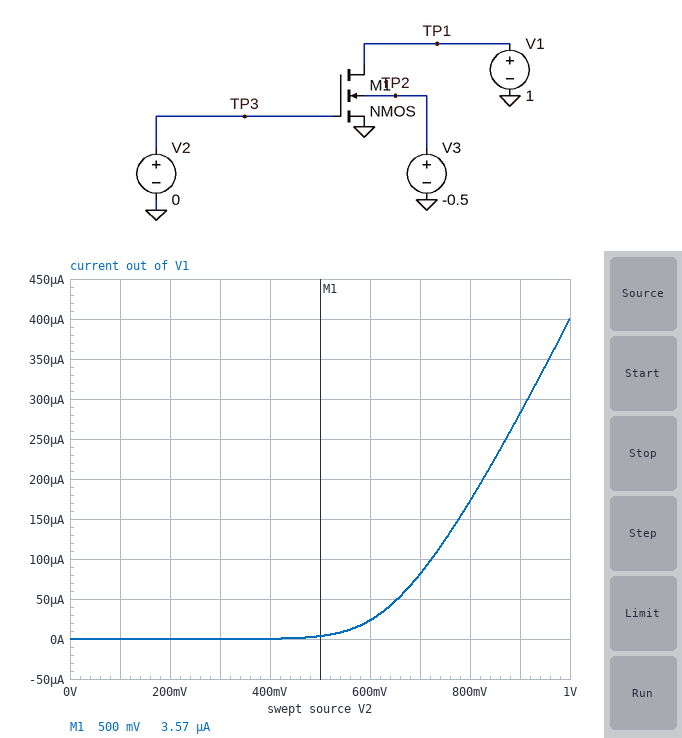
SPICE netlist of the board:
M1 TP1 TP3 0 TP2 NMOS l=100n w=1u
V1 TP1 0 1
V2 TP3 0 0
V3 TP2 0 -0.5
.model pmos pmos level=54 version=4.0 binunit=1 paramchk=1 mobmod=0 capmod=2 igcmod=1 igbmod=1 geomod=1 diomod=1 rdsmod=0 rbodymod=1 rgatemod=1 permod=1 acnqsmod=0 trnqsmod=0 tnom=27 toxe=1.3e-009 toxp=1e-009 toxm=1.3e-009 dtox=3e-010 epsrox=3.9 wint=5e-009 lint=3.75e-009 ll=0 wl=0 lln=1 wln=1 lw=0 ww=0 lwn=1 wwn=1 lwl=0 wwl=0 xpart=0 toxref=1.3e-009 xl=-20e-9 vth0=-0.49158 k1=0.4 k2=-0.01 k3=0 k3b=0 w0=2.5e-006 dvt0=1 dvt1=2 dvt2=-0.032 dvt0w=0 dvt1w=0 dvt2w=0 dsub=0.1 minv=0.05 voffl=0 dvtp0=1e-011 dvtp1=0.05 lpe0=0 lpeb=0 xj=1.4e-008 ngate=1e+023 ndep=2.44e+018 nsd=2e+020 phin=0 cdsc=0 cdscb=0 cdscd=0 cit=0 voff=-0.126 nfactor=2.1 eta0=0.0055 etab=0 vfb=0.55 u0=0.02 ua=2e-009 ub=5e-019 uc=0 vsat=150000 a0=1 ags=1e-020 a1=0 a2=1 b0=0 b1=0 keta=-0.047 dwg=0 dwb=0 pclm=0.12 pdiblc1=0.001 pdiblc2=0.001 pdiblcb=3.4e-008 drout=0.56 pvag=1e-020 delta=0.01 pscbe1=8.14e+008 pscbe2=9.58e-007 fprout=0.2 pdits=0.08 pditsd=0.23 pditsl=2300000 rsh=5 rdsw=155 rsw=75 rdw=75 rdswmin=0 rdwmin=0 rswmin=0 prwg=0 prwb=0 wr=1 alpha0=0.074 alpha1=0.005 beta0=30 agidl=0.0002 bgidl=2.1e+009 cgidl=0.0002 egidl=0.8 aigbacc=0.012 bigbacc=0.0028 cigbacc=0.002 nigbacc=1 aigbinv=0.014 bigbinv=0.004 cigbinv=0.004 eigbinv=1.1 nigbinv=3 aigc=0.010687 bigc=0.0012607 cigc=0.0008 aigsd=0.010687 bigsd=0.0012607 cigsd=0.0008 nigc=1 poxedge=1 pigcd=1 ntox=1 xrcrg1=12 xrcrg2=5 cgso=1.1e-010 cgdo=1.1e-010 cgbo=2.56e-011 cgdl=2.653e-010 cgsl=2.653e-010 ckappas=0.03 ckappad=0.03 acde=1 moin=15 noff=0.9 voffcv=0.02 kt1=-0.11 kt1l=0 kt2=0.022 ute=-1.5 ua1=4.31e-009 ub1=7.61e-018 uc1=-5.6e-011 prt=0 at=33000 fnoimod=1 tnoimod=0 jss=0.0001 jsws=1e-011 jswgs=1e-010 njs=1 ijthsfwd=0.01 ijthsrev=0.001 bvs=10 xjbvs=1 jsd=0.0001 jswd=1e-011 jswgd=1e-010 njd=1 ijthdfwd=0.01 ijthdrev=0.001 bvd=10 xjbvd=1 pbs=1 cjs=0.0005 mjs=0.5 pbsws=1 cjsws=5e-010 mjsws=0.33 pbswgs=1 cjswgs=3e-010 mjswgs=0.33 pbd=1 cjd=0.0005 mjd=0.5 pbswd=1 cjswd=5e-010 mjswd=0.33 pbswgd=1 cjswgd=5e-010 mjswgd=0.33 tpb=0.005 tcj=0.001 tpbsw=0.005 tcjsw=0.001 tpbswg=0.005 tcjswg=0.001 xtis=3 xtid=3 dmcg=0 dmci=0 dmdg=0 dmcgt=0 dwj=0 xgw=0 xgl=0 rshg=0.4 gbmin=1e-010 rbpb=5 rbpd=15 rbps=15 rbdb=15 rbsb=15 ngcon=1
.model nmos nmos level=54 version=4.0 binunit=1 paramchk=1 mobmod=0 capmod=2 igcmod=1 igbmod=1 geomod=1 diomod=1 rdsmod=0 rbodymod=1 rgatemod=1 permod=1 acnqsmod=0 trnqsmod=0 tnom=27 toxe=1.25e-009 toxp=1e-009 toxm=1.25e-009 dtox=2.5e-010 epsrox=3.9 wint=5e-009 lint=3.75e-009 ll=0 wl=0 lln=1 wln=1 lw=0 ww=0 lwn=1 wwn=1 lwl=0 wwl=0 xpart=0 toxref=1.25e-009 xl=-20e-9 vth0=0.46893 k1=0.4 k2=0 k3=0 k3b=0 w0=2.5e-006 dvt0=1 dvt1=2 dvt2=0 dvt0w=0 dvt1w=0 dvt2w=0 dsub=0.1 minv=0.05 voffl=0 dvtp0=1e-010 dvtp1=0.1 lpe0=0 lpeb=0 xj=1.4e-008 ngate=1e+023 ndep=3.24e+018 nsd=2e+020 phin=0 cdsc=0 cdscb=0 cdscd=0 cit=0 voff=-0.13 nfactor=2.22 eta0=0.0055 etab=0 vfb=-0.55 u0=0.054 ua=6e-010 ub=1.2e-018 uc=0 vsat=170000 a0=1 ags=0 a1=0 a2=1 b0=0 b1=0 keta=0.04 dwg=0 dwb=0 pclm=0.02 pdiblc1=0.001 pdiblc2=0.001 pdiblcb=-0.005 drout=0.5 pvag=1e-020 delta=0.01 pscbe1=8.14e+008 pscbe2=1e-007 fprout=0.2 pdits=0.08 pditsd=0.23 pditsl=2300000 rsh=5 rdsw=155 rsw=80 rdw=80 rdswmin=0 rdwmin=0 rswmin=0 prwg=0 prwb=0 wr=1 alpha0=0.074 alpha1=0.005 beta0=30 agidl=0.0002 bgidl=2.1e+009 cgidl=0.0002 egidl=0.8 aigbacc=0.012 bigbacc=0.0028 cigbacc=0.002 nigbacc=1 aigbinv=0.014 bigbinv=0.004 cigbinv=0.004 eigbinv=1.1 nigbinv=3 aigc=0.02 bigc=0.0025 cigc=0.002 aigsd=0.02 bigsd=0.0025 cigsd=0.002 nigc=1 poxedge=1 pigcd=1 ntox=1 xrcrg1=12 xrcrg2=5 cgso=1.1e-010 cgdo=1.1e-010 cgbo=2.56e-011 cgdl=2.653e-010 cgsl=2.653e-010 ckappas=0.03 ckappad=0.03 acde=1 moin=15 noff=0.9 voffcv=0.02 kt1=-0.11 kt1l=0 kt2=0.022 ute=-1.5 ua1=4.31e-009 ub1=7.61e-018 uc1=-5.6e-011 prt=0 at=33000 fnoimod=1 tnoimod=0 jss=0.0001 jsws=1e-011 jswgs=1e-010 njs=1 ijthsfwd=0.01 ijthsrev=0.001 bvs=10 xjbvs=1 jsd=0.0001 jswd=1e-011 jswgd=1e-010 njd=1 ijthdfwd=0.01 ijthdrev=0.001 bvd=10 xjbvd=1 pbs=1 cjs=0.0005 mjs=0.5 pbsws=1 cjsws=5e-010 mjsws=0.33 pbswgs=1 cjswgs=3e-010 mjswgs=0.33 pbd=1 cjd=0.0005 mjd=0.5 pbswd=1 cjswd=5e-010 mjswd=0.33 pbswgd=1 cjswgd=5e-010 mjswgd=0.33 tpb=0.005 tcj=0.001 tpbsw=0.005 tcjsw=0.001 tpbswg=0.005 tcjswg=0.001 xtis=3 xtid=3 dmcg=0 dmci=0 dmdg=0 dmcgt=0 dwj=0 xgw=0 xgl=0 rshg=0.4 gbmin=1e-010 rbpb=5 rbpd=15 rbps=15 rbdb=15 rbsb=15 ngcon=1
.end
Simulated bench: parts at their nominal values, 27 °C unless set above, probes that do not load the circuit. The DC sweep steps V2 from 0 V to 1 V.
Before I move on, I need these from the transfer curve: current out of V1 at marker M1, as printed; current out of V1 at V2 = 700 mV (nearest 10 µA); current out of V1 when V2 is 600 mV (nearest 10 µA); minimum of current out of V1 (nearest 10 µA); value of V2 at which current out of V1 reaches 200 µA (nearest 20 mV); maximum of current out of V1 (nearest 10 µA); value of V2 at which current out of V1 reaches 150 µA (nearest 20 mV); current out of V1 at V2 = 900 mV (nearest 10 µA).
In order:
3.57 µA
80 µA
20 µA
0 A
820 mV
400 µA
780 mV
280 µA
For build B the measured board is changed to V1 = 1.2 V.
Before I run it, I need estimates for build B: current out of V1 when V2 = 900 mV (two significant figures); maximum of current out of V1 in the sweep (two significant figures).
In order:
290 µA
410 µA
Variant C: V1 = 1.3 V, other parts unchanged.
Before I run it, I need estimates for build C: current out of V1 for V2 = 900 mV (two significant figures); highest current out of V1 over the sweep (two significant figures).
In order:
290 µA
410 µA
